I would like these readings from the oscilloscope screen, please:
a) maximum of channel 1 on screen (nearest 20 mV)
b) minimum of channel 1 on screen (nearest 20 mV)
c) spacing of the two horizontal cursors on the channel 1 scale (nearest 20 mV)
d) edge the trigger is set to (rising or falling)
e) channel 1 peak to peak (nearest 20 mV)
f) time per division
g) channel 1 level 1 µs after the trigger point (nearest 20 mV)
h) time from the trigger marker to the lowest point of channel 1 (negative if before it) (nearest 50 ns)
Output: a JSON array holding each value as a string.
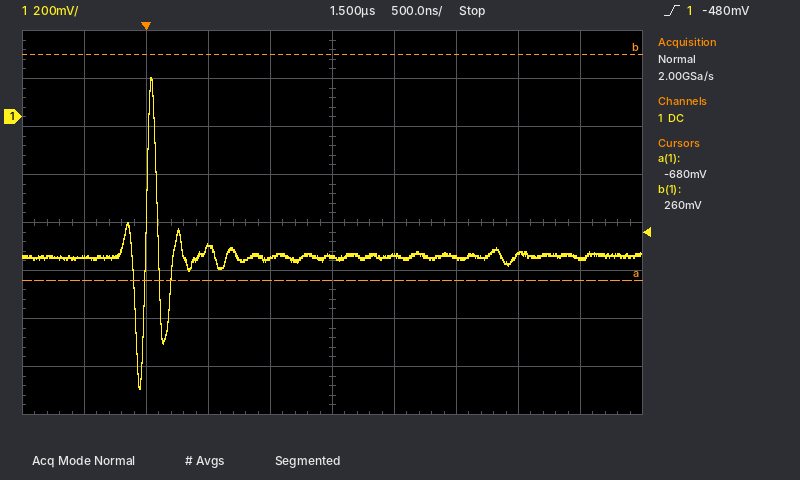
["160 mV", "-1.14 V", "940 mV", "rising", "1.30 V", "500 ns", "-580 mV", "-50 ns"]
